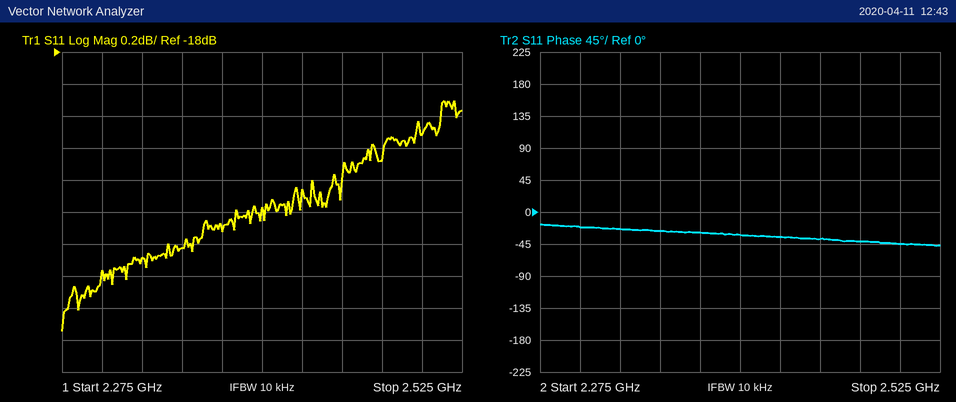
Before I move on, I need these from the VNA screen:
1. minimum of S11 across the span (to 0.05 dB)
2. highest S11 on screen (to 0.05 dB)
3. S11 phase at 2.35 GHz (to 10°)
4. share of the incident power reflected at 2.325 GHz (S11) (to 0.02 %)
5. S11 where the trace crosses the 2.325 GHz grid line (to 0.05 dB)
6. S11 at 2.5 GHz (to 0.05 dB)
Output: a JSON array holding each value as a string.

["-19.75 dB", "-18.30 dB", "-30°", "1.18 %", "-19.30 dB", "-18.50 dB"]
